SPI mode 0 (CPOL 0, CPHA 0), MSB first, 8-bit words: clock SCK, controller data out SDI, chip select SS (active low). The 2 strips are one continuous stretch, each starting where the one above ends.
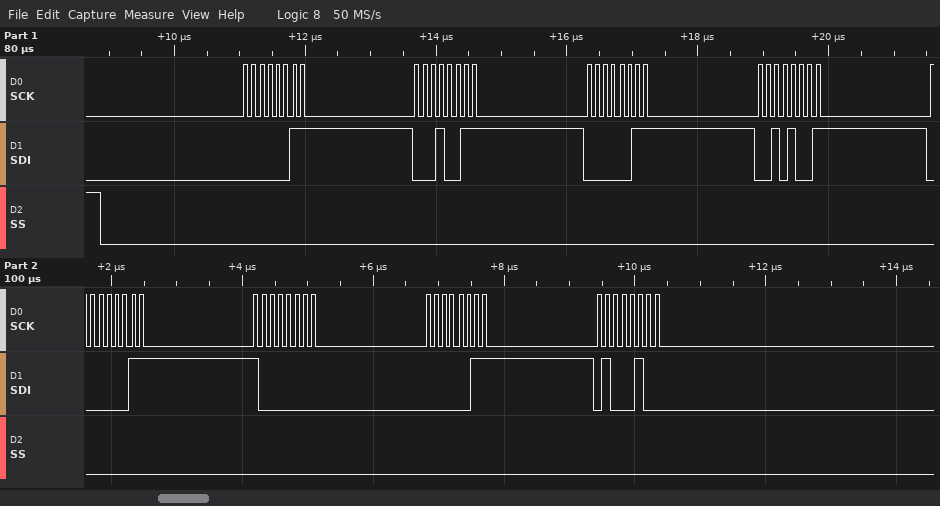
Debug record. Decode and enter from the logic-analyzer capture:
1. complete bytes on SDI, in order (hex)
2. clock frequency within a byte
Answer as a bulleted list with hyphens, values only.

- 03 13 03 29 03 80 03 44
- 8 MHz
